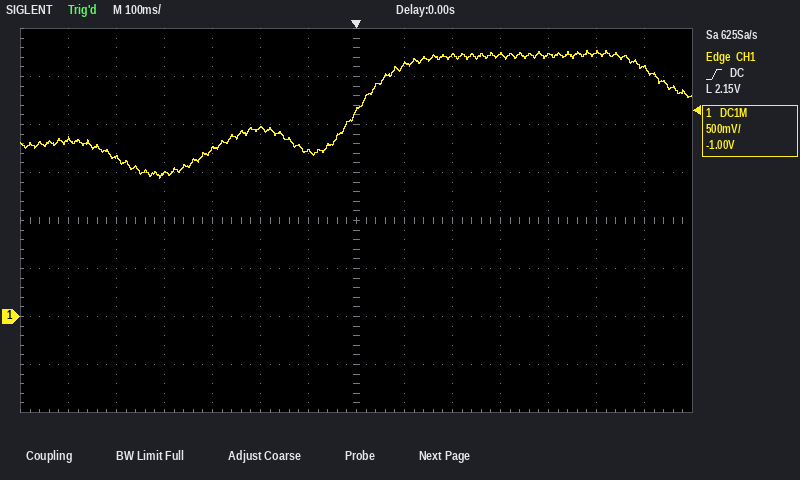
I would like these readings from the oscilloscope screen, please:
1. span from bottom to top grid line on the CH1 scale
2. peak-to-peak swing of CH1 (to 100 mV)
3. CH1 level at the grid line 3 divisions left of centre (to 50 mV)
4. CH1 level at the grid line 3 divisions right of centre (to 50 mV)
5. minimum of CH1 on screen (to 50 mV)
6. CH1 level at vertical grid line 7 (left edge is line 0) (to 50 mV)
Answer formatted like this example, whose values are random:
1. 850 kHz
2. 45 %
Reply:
1. 4 V
2. 1.30 V
3. 1.75 V
4. 2.75 V
5. 1.45 V
6. 2.15 V
